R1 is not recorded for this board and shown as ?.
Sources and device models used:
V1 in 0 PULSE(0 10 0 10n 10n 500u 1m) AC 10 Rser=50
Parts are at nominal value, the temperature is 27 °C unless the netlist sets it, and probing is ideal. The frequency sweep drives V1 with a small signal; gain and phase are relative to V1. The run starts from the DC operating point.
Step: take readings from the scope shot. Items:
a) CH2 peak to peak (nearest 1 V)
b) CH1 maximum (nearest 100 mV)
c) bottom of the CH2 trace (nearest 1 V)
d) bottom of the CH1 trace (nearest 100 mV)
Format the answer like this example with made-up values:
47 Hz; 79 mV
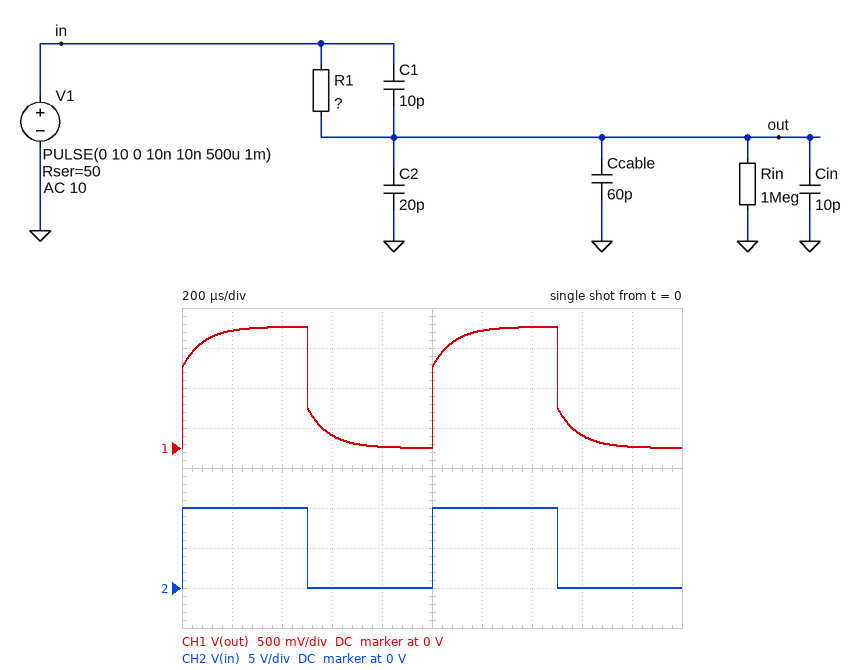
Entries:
10 V; 1.5 V; 0 V; 0 V
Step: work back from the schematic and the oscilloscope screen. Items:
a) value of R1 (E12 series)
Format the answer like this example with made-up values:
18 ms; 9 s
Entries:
5.6 MΩ
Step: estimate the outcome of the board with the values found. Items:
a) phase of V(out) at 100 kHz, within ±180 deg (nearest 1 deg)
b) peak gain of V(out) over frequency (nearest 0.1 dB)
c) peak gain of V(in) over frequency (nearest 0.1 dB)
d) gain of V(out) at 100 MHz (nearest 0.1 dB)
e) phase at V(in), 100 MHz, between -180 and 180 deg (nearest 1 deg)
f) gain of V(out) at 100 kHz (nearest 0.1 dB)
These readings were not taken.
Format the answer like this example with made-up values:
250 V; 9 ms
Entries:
-1 deg; -16.4 dB; 0 dB; -20.3 dB; -16 deg; -20.0 dB
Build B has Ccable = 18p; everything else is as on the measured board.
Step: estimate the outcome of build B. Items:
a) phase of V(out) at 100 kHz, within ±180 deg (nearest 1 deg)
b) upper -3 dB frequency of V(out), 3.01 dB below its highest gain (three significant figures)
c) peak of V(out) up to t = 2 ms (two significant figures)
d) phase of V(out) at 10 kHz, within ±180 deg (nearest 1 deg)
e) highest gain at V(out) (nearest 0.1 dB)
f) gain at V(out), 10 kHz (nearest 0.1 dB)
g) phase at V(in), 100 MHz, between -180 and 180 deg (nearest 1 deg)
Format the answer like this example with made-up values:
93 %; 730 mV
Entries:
0 deg; 385 MHz; 1.7 V; 2 deg; -15.3 dB; -15.4 dB; -15 deg
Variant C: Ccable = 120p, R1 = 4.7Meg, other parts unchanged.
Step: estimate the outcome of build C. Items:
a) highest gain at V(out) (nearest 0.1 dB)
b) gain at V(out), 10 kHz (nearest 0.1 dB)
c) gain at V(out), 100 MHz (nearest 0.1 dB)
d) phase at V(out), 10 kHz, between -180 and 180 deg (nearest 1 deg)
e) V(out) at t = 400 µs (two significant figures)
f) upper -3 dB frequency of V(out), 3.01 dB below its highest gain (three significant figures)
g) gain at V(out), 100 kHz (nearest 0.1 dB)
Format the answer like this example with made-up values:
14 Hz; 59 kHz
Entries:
-15.1 dB; -23.7 dB; -24.4 dB; -12 deg; 1.7 V; 1.40 kHz; -24.1 dB
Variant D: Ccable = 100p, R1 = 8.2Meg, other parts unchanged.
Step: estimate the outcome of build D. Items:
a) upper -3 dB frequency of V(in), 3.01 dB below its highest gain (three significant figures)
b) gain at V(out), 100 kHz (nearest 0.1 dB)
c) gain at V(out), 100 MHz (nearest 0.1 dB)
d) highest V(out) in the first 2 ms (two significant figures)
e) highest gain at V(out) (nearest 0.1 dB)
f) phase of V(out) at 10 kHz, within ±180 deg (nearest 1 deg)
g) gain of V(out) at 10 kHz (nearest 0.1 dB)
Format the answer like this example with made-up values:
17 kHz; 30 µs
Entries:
343 MHz; -22.9 dB; -23.3 dB; 1.1 V; -19.3 dB; -4 deg; -22.8 dB
